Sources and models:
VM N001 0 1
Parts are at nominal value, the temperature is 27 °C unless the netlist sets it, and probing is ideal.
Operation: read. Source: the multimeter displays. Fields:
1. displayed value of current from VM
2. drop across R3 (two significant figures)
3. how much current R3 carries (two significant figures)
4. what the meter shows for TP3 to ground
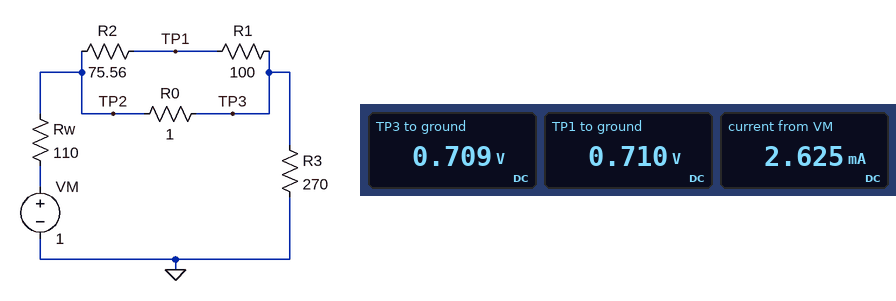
2.625 mA
710 mV
2.6 mA
0.709 V
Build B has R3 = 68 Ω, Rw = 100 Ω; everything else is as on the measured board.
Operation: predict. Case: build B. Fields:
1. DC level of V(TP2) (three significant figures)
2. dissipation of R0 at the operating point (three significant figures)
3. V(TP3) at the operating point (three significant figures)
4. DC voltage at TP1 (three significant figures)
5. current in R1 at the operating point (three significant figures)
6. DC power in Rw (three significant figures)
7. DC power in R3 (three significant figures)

408 mV
34.6 µW
402 mV
406 mV
33.5 µA
3.50 mW
2.38 mW
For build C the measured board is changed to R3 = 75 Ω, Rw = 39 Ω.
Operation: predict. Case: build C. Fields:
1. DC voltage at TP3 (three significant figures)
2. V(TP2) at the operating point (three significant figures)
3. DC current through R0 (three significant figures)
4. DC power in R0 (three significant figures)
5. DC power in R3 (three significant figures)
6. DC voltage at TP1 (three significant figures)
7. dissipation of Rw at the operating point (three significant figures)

652 mV
661 mV
8.65 mA
74.8 µW
5.67 mW
657 mV
2.95 mW
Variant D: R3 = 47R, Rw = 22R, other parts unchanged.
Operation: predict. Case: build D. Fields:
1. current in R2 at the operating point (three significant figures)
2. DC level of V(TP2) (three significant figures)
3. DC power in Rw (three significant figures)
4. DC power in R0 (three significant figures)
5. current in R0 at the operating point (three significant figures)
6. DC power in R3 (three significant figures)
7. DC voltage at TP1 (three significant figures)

80.9 µA
686 mV
4.49 mW
202 µW
14.2 mA
9.59 mW
680 mV
